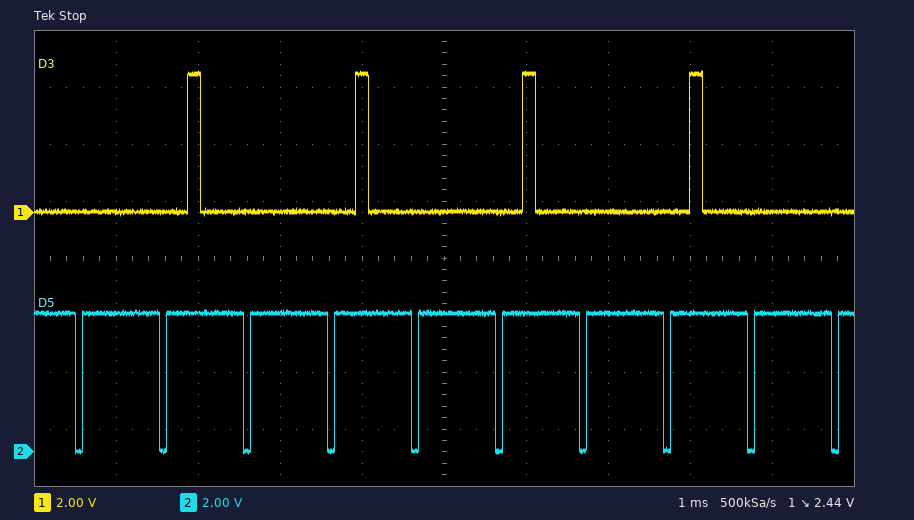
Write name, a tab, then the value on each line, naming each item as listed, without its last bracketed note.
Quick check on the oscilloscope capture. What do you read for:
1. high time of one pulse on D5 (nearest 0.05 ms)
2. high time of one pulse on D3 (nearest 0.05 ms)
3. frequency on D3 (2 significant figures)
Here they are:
high time of one pulse on D5	0.95 ms
high time of one pulse on D3	0.15 ms
frequency on D3	490 Hz
